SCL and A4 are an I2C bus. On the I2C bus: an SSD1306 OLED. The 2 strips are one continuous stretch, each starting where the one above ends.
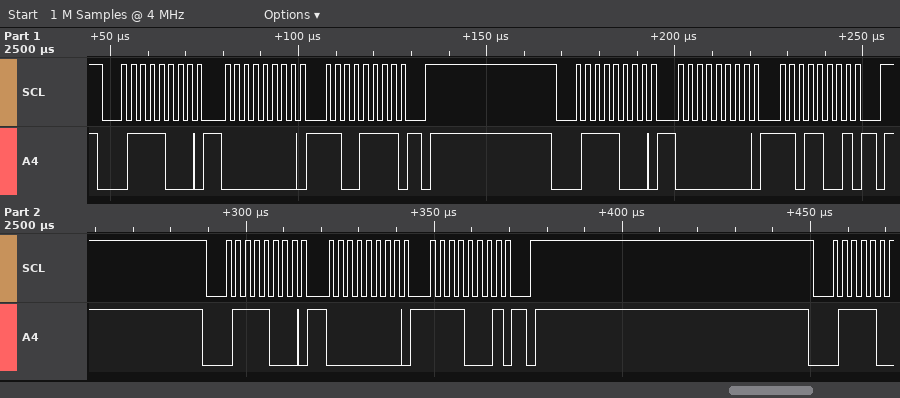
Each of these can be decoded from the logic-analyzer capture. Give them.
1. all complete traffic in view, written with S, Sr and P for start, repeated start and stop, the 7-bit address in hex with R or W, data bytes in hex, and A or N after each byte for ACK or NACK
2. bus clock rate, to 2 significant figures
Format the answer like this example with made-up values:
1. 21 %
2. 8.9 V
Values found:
1. S 3CW A 00 A CF A P S 3CW A 00 A D9 A P S 3CW A 00 A F1 A P
2. 400 kHz
